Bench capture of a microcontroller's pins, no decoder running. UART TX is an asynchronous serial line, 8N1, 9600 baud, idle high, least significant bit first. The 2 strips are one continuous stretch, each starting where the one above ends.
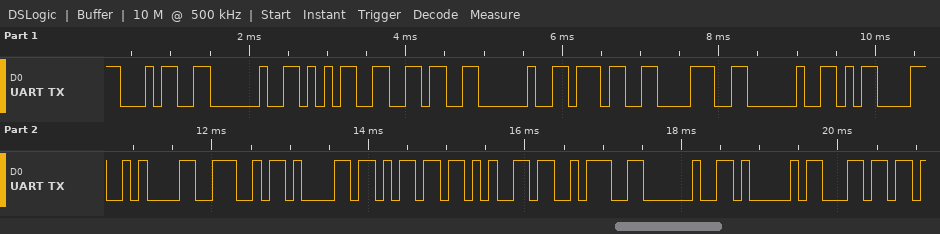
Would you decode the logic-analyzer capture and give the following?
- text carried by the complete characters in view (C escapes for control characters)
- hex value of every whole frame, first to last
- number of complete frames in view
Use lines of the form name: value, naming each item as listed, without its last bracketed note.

text carried by the complete characters in view: "4 56 78 \r\nName: Al"
hex value of every whole frame, first to last: 34 20 35 36 20 37 38 20 0D 0A 4E 61 6D 65 3A 20 41 6C
number of complete frames in view: 18
